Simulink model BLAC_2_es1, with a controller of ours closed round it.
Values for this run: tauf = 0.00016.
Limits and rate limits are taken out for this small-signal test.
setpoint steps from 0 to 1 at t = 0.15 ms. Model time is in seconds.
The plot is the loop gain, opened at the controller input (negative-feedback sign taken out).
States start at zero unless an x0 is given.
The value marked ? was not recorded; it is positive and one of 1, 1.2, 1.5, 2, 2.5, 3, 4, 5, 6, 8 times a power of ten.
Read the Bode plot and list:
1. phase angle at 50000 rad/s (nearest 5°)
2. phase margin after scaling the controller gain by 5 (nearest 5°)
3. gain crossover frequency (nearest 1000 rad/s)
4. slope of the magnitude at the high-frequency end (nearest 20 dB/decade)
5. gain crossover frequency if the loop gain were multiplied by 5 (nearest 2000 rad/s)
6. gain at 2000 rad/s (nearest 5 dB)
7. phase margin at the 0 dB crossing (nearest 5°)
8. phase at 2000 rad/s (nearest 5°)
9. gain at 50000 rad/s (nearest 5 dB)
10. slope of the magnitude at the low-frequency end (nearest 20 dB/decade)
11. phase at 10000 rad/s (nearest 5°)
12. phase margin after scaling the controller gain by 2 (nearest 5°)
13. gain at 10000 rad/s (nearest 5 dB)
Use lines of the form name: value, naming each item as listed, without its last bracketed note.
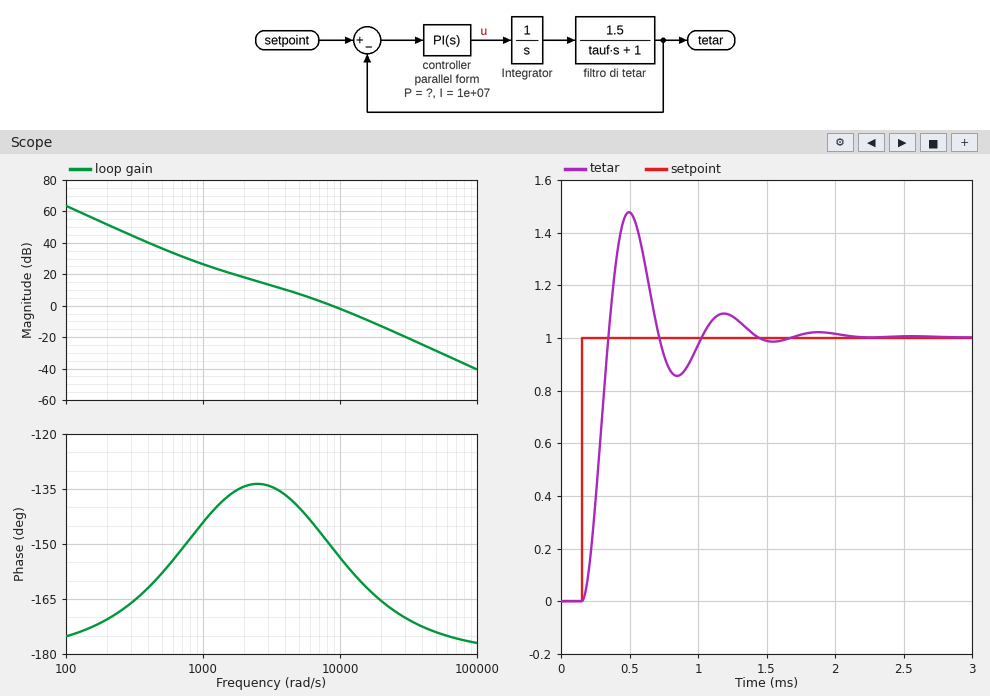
phase angle at 50000 rad/s: -175°
phase margin after scaling the controller gain by 5: 15°
gain crossover frequency: 9000 rad/s
slope of the magnitude at the high-frequency end: -40 dB/decade
gain crossover frequency if the loop gain were multiplied by 5: 22000 rad/s
gain at 2000 rad/s: 20 dB
phase margin at the 0 dB crossing: 30°
phase at 2000 rad/s: -135°
gain at 50000 rad/s: -30 dB
slope of the magnitude at the low-frequency end: -40 dB/decade
phase at 10000 rad/s: -155°
phase margin after scaling the controller gain by 2: 20°
gain at 10000 rad/s: 0 dB
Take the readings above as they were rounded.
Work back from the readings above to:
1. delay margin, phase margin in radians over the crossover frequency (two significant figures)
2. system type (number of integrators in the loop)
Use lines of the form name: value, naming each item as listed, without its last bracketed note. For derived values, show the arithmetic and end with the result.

delay margin, phase margin in radians over the crossover frequency: 30 × π / 180 / 9000 = 0.000058 s
system type: 2
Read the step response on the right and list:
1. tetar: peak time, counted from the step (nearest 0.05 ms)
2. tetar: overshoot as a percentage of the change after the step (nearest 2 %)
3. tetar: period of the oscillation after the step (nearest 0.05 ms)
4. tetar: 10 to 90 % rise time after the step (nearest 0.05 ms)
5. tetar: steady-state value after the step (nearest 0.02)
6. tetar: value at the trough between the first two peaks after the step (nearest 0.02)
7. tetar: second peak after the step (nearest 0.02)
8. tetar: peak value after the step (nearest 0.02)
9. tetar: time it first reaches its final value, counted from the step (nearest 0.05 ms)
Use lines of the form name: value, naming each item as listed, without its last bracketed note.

tetar: peak time, counted from the step: 0.35 ms
tetar: overshoot as a percentage of the change after the step: 48 %
tetar: period of the oscillation after the step: 0.70 ms
tetar: 10 to 90 % rise time after the step: 0.15 ms
tetar: steady-state value after the step: 1.00
tetar: value at the trough between the first two peaks after the step: 0.86
tetar: second peak after the step: 1.10
tetar: peak value after the step: 1.48
tetar: time it first reaches its final value, counted from the step: 0.20 ms
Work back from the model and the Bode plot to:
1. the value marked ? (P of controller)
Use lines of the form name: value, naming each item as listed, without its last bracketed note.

the value marked ?: 10000
